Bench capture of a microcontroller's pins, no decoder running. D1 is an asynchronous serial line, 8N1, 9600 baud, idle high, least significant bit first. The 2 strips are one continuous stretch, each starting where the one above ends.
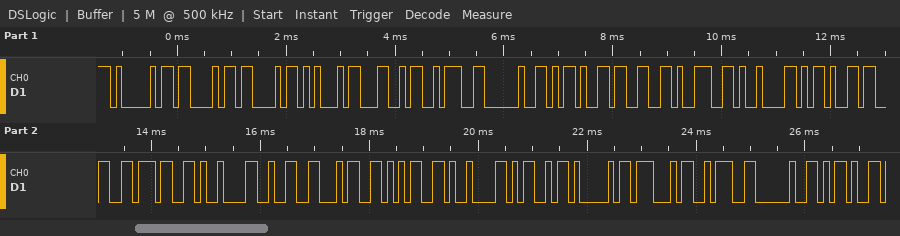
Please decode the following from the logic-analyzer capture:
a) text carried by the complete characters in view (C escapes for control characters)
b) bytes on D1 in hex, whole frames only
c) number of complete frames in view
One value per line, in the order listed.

"ACCEL: -39\t-37\t245\tMAG: -"
41 43 43 45 4C 3A 20 2D 33 39 09 2D 33 37 09 32 34 35 09 4D 41 47 3A 20 2D
25
